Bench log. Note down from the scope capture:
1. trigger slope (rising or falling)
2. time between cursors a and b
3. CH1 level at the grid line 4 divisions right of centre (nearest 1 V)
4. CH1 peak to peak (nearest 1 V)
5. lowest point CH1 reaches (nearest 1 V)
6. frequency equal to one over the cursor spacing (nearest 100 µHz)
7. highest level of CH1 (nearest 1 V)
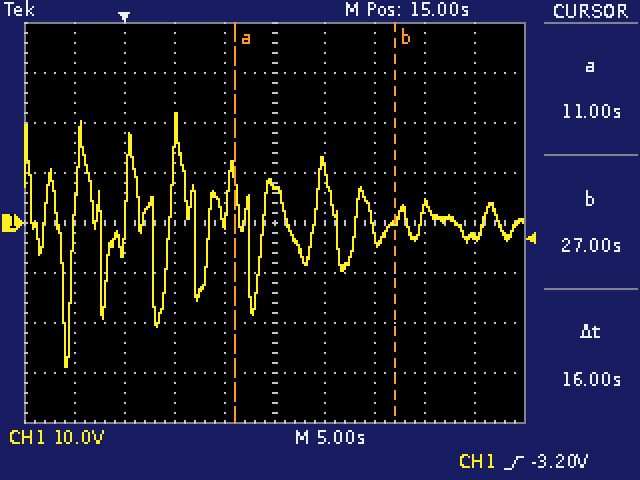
rising
16 s
-3 V
51 V
-29 V
62.5 mHz
22 V
